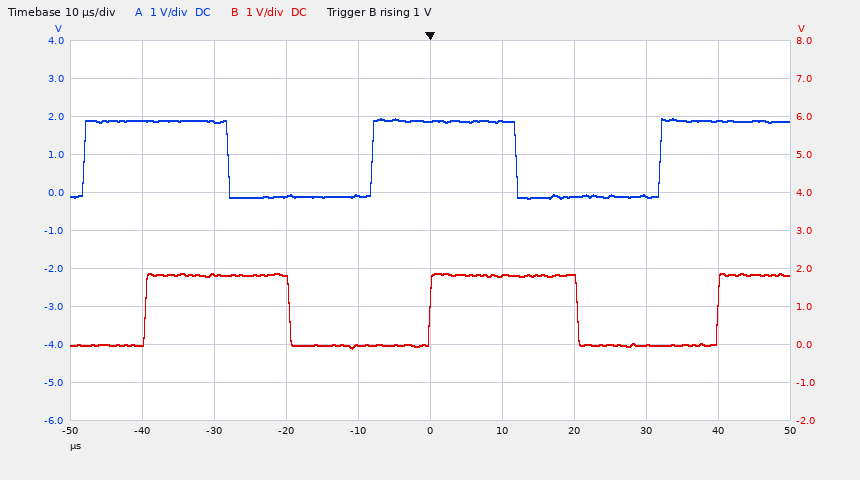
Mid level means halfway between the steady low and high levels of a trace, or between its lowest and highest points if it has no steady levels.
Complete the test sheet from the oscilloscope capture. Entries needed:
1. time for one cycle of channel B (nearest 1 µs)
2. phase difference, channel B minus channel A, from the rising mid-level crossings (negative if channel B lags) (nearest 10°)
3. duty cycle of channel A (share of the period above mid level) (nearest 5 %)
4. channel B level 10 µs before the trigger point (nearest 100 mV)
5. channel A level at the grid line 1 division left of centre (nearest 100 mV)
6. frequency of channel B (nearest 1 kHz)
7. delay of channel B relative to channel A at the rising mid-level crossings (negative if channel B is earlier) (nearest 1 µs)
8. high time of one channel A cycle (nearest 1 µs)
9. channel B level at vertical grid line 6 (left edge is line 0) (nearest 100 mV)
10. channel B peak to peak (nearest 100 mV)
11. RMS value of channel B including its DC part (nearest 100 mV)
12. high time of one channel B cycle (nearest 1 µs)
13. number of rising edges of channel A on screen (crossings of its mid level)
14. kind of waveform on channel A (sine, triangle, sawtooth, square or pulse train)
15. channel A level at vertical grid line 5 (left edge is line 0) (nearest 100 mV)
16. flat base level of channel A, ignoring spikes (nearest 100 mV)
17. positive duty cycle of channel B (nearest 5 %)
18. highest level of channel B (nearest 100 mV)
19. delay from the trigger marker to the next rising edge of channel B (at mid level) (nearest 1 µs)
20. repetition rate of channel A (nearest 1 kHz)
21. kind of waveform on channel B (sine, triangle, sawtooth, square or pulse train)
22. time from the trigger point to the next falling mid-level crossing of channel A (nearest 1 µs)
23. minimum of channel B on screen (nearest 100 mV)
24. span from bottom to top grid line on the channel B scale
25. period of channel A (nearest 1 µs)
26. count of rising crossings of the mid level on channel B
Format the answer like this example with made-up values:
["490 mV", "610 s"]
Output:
["40 µs", "-70°", "50 %", "0.0 V", "-100 mV", "25 kHz", "+8 µs", "20 µs", "1.8 V", "2.0 V", "1.3 V", "20 µs", "3", "square", "1.9 V", "-100 mV", "50 %", "1.9 V", "40 µs", "25 kHz", "square", "12 µs", "-100 mV", "10 V", "40 µs", "3"]
